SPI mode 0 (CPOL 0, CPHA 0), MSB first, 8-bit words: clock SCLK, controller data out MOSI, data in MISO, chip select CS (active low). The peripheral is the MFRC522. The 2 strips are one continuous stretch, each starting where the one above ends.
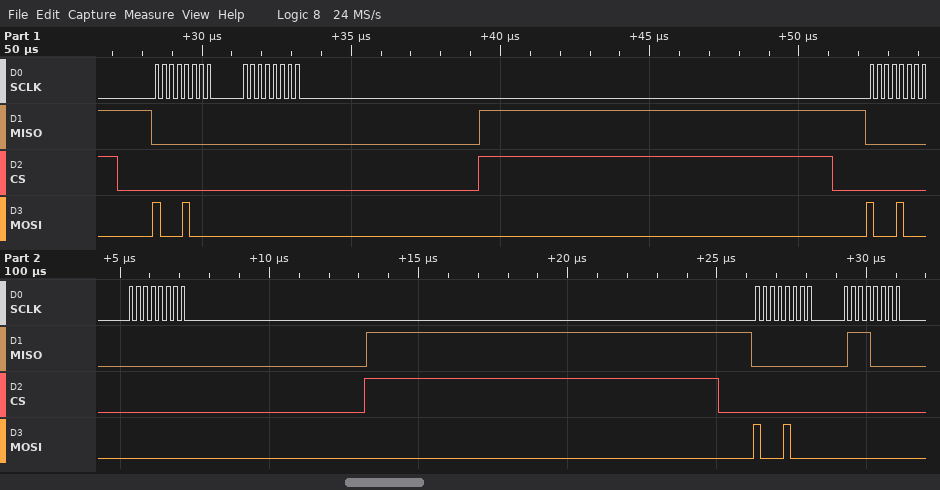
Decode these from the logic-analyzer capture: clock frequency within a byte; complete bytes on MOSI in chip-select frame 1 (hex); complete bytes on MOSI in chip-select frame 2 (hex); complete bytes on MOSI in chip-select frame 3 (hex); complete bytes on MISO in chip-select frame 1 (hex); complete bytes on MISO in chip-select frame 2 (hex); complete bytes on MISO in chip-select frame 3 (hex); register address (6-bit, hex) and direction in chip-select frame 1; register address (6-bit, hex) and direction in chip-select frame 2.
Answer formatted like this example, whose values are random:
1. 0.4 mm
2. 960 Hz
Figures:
1. 4 MHz
2. 88 00
3. 88 00
4. 88 00
5. 00 00
6. 00 00
7. 00 70
8. 0x04 read
9. 0x04 read
